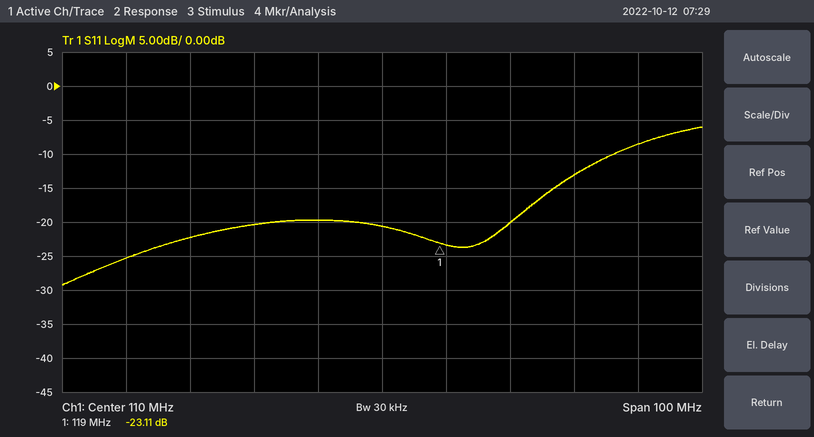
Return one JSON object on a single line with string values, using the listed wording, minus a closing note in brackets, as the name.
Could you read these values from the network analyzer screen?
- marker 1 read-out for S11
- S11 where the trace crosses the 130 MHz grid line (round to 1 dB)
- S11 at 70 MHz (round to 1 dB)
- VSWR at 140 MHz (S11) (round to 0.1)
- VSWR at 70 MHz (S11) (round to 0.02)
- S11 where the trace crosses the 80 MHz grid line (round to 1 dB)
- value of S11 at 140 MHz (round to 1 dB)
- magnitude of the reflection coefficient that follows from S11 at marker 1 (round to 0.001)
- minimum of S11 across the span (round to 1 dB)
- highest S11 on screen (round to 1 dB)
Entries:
{"marker 1 read-out for S11": "-23.11 dB", "S11 where the trace crosses the 130 MHz grid line": "-20 dB", "S11 at 70 MHz": "-25 dB", "VSWR at 140 MHz (S11)": "1.6", "VSWR at 70 MHz (S11)": "1.12", "S11 where the trace crosses the 80 MHz grid line": "-22 dB", "value of S11 at 140 MHz": "-13 dB", "magnitude of the reflection coefficient that follows from S11 at marker 1": "0.070", "minimum of S11 across the span": "-29 dB", "highest S11 on screen": "-6 dB"}
